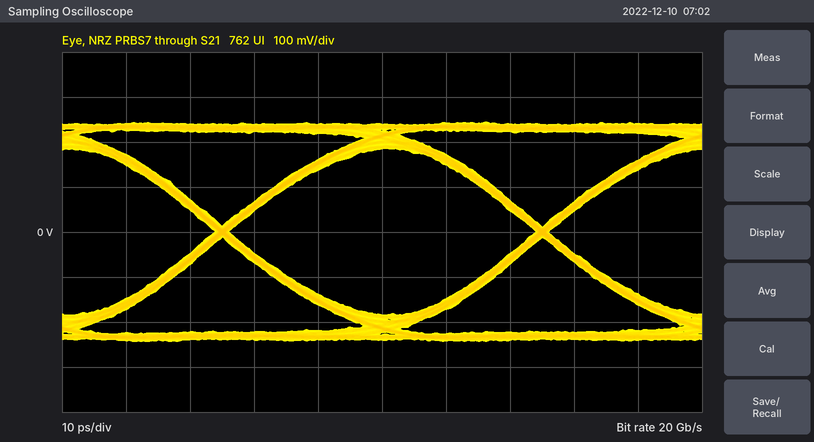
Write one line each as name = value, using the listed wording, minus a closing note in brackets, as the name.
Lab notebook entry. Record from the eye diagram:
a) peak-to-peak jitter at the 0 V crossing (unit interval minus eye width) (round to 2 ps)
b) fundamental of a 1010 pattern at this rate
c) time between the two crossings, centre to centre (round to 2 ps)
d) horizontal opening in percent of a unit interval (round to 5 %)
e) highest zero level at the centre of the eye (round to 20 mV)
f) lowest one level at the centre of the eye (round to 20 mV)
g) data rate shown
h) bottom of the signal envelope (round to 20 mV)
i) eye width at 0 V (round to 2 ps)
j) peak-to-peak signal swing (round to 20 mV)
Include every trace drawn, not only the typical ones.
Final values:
peak-to-peak jitter at the 0 V crossing (unit interval minus eye width) = 2 ps
fundamental of a 1010 pattern at this rate = 10 GHz
time between the two crossings, centre to centre = 50 ps
horizontal opening in percent of a unit interval = 95 %
highest zero level at the centre of the eye = -180 mV
lowest one level at the centre of the eye = 180 mV
data rate shown = 20 Gb/s
bottom of the signal envelope = -240 mV
eye width at 0 V = 48 ps
peak-to-peak signal swing = 480 mV
